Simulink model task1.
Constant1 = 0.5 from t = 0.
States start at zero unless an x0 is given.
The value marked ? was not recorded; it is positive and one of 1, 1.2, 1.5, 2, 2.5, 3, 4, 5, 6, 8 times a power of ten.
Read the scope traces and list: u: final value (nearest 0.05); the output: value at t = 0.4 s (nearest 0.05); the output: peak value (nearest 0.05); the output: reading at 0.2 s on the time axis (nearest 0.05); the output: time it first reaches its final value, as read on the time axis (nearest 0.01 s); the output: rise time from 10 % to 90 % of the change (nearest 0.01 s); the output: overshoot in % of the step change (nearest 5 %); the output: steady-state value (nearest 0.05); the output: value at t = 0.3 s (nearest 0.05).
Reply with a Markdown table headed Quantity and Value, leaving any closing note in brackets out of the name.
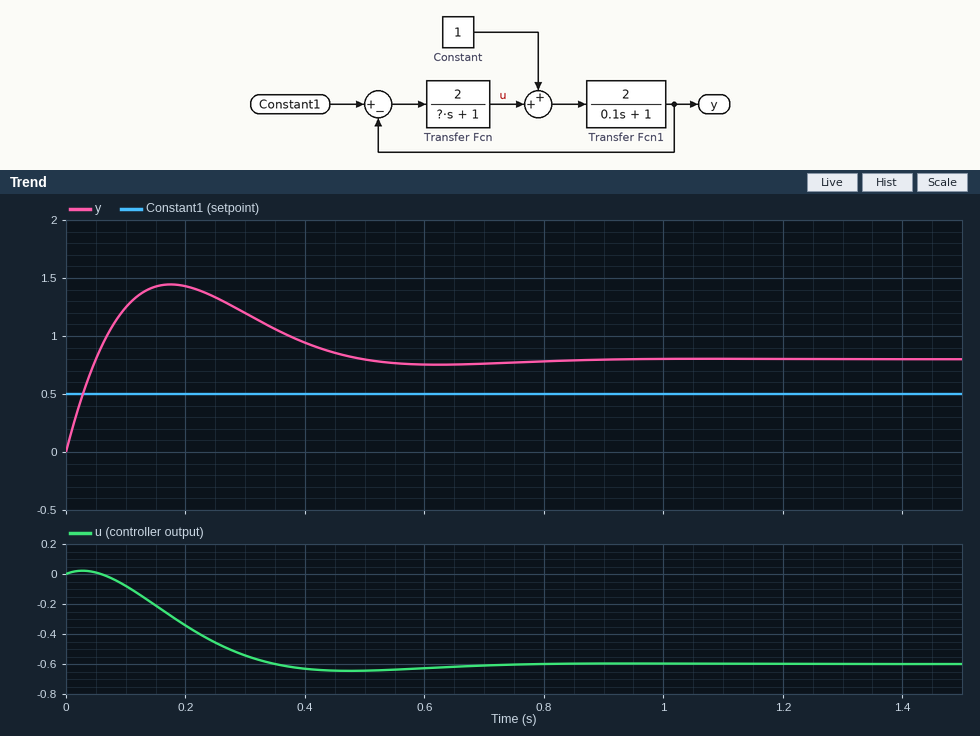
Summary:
| Quantity | Value |
|---|---|
| u: final value | -0.60 |
| the output: value at t = 0.4 s | 0.95 |
| the output: peak value | 1.45 |
| the output: reading at 0.2 s on the time axis | 1.45 |
| the output: time it first reaches its final value, as read on the time axis | 0.05 s |
| the output: rise time from 10 % to 90 % of the change | 0.04 s |
| the output: overshoot in % of the step change | 80 % |
| the output: steady-state value | 0.80 |
| the output: value at t = 0.3 s | 1.20 |
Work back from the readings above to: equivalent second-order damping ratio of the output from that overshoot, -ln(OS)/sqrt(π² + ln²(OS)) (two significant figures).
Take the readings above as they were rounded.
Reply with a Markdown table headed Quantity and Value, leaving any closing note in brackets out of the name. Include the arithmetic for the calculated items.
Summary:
| Quantity | Value |
|---|---|
| equivalent second-order damping ratio of the output from that overshoot, -ln(OS)/sqrt(π² + ln²(OS)) | ln(0.8) = -0.223; 0.223 / sqrt(9.870 + 0.050) = 0.071 |
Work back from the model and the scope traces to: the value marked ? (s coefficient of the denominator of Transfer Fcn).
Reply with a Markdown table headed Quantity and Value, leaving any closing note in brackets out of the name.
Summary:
| Quantity | Value |
|---|---|
| the value marked ? | 0.6 |
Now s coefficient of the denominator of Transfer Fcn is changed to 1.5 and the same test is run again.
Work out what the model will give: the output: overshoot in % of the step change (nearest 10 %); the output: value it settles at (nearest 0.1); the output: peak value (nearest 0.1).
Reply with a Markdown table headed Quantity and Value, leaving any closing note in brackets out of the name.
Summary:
| Quantity | Value |
|---|---|
| the output: overshoot in % of the step change | 100 % |
| the output: value it settles at | 0.8 |
| the output: peak value | 1.6 |
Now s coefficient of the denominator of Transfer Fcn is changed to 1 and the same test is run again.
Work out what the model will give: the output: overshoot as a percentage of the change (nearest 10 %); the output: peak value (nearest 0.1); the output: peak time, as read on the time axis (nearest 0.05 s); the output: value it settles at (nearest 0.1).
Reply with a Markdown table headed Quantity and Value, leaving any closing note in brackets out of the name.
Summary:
| Quantity | Value |
|---|---|
| the output: overshoot as a percentage of the change | 90 % |
| the output: peak value | 1.5 |
| the output: peak time, as read on the time axis | 0.20 s |
| the output: value it settles at | 0.8 |
